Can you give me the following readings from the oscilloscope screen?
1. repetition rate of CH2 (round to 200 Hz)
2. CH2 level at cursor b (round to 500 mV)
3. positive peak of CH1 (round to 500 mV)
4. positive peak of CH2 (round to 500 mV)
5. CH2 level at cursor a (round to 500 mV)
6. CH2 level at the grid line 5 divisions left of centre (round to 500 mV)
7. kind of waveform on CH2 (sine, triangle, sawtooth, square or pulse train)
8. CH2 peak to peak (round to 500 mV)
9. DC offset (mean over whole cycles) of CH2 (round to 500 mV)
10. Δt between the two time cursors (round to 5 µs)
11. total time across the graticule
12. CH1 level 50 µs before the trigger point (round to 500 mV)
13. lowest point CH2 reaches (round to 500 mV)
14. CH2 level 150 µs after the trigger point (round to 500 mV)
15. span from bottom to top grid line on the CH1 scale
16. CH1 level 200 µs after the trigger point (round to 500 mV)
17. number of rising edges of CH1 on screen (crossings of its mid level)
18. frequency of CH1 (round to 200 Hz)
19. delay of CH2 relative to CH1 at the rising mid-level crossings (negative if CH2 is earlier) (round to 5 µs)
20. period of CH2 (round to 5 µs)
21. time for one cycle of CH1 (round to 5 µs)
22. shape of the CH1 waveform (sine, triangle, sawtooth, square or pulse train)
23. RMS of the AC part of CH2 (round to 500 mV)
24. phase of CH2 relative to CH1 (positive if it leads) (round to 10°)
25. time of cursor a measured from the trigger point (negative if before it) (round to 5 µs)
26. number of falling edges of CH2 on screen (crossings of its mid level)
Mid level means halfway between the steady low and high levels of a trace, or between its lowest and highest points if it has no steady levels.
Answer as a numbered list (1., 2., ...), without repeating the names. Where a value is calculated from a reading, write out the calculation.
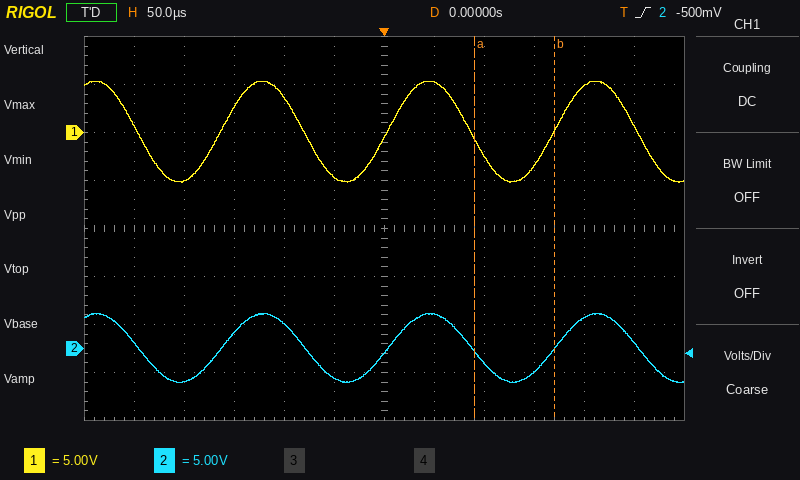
1. 1 / 165 µs ≈ 6.06 kHz, so 6.0 kHz to the nearest 200 Hz
2. 0.0 V
3. 5.5 V
4. 3.5 V
5. -500 mV
6. 500 mV
7. sine
8. 3.5 V − (-3.5 V) = 7.0 V
9. (3.5 V + (-3.5 V)) / 2 ≈ 0.0 V
10. 80 µs
11. 600 µs
12. -4.5 V
13. -3.5 V
14. -2.5 V
15. 40 V
16. 5.0 V
17. 3
18. 1 / 165 µs ≈ 6.06 kHz, so 6.0 kHz to the nearest 200 Hz
19. 0 µs
20. 165 µs
21. 165 µs
22. sine
23. 7.0 V / (2√2) ≈ 2.5 V
24. −360° × (0 µs) / 165 µs ≈ 0°
25. +90 µs
26. 4
